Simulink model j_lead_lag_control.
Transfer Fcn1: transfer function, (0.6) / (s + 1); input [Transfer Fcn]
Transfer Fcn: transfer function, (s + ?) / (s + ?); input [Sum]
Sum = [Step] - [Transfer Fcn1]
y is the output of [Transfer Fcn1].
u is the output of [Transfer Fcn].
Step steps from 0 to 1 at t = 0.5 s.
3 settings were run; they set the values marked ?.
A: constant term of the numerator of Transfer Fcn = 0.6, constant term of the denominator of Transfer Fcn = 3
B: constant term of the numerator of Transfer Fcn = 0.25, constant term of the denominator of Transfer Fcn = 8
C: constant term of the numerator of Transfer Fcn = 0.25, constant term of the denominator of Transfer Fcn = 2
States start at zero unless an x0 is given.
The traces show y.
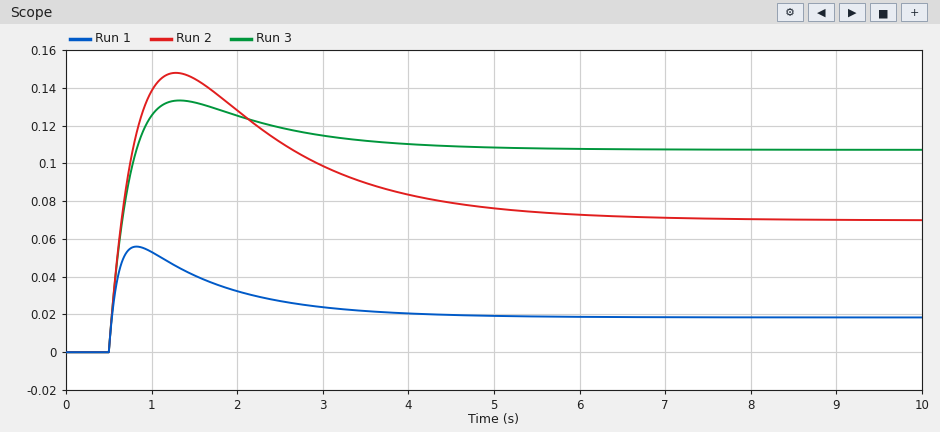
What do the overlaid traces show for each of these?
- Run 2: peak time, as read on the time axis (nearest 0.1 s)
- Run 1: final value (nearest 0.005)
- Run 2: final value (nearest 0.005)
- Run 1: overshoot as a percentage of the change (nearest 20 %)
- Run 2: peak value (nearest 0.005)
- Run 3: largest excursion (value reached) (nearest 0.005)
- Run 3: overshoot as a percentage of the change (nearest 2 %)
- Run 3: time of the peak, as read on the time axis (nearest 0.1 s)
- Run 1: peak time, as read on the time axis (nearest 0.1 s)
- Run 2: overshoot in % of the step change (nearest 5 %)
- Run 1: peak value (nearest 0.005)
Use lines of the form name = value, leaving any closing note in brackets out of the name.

Run 2: peak time, as read on the time axis = 1.3 s
Run 1: final value = 0.020
Run 2: final value = 0.070
Run 1: overshoot as a percentage of the change = 200 %
Run 2: peak value = 0.150
Run 3: largest excursion (value reached) = 0.135
Run 3: overshoot as a percentage of the change = 24 %
Run 3: time of the peak, as read on the time axis = 1.3 s
Run 1: peak time, as read on the time axis = 0.8 s
Run 2: overshoot in % of the step change = 110 %
Run 1: peak value = 0.055
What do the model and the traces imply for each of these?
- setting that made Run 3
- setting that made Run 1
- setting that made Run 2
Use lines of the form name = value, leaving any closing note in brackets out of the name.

setting that made Run 3 = A
setting that made Run 1 = B
setting that made Run 2 = C
